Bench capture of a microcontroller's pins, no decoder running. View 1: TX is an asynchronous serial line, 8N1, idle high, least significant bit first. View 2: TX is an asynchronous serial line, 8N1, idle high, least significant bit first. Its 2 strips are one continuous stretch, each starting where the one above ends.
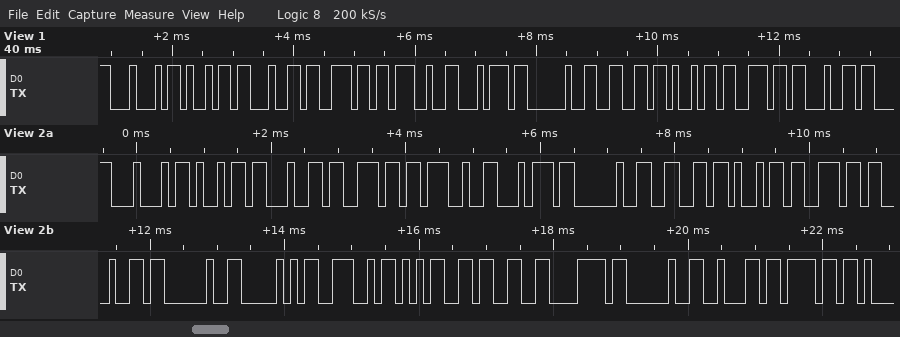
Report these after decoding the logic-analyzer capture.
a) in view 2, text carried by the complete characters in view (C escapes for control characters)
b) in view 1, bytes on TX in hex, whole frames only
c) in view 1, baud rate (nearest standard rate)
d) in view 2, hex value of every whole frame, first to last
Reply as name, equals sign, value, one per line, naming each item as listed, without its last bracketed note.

in view 2, text carried by the complete characters in view = "Didn't find PN53x bo"
in view 1, bytes on TX in hex, whole frames only = 44 69 64 6E 27 74 20 66 69 6E 64
in view 1, baud rate = 9600 baud
in view 2, hex value of every whole frame, first to last = 0x44 0x69 0x64 0x6E 0x27 0x74 0x20 0x66 0x69 0x6E 0x64 0x20 0x50 0x4E 0x35 0x33 0x78 0x20 0x62 0x6F
